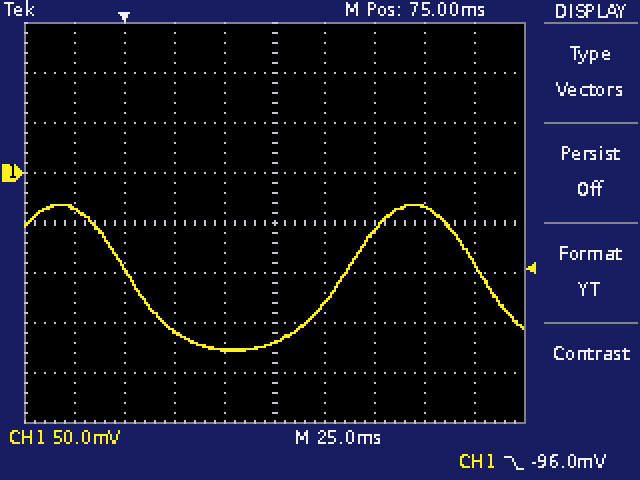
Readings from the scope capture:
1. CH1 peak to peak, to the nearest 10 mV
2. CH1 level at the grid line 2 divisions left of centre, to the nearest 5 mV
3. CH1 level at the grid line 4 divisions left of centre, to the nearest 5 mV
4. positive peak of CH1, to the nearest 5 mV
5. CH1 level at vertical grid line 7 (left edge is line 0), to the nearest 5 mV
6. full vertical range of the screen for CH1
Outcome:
150 mV
-160 mV
-35 mV
-30 mV
-60 mV
400 mV
